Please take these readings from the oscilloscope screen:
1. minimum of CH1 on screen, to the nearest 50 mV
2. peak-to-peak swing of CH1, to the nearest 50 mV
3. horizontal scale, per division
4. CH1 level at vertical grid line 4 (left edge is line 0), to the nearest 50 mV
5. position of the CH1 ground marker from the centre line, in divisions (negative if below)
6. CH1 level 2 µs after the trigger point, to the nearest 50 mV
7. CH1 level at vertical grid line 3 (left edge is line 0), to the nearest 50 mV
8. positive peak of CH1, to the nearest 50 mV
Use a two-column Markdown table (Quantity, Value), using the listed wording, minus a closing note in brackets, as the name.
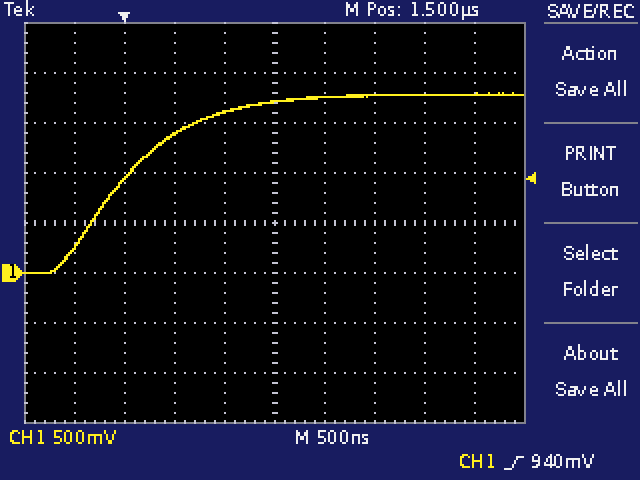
| Quantity | Value |
|---|---|
| minimum of CH1 on screen, to the nearest 50 mV | 0 mV |
| peak-to-peak swing of CH1, to the nearest 50 mV | 1.80 V |
| horizontal scale, per division | 500 ns |
| CH1 level at vertical grid line 4 (left edge is line 0), to the nearest 50 mV | 1.60 V |
| position of the CH1 ground marker from the centre line, in divisions | -1.0 div |
| CH1 level 2 µs after the trigger point, to the nearest 50 mV | 1.75 V |
| CH1 level at vertical grid line 3 (left edge is line 0), to the nearest 50 mV | 1.40 V |
| positive peak of CH1, to the nearest 50 mV | 1.80 V |
